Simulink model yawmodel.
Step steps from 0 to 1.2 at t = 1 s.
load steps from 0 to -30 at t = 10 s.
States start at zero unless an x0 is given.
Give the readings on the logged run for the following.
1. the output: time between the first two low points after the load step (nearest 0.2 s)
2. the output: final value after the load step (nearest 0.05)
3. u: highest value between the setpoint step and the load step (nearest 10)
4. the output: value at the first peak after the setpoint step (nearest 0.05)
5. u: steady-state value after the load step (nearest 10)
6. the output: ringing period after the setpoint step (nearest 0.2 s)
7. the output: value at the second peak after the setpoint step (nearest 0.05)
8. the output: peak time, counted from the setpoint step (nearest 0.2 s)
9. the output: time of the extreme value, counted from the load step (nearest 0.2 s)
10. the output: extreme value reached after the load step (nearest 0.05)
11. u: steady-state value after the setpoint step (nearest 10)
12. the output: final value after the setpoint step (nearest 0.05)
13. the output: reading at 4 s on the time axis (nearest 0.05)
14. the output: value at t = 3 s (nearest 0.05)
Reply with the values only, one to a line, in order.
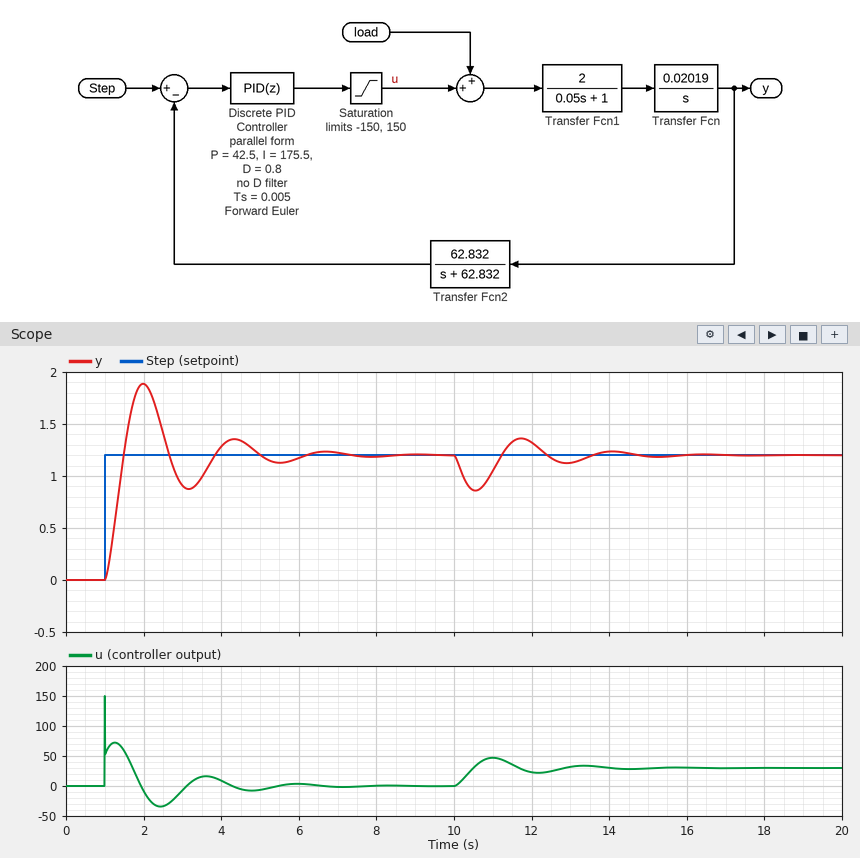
2.4 s
1.20
150
1.90
30
2.4 s
1.35
1.0 s
0.6 s
0.85
0
1.20
1.30
0.90
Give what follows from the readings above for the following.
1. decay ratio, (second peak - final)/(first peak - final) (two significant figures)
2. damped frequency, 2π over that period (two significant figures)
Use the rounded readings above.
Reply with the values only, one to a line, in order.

0.21
2.6 rad/s
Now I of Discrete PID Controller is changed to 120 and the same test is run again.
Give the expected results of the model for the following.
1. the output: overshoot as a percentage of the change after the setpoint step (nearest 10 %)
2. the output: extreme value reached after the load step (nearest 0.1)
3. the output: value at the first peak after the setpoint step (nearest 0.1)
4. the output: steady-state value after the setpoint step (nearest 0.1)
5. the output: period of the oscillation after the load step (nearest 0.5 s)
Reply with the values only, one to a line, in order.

50 %
0.8
1.8
1.2
3.0 s
